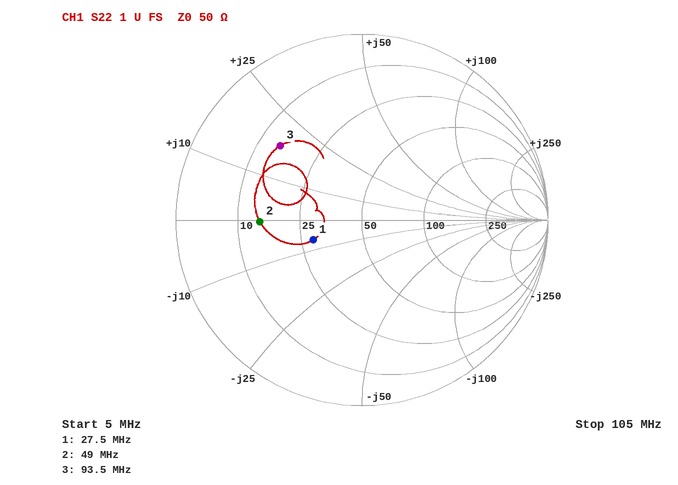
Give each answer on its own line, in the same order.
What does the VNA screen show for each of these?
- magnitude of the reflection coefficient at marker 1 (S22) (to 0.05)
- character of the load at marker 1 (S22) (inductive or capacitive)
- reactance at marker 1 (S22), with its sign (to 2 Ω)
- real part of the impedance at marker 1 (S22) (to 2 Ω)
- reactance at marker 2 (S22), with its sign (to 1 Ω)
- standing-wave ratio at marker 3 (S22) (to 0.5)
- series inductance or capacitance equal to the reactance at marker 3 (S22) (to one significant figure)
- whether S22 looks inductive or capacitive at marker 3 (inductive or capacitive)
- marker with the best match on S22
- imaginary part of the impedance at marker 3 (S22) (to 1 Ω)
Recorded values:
0.30
capacitive
-6 Ω
28 Ω
0 Ω
4.0
30 nH
inductive
marker 1
+18 Ω
